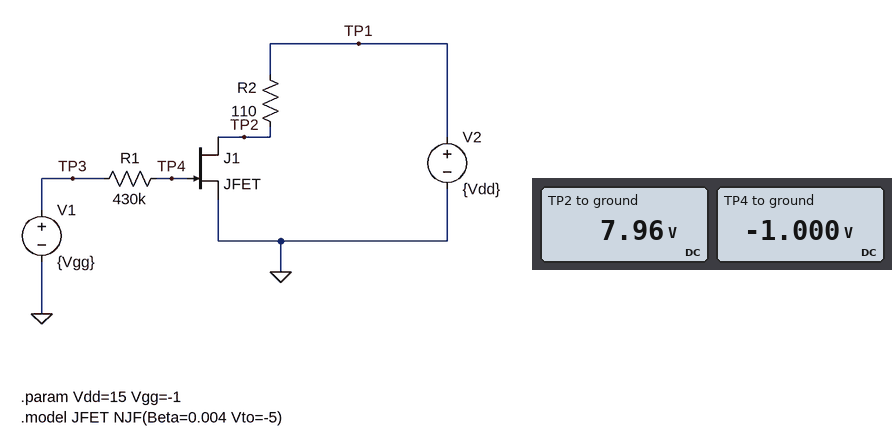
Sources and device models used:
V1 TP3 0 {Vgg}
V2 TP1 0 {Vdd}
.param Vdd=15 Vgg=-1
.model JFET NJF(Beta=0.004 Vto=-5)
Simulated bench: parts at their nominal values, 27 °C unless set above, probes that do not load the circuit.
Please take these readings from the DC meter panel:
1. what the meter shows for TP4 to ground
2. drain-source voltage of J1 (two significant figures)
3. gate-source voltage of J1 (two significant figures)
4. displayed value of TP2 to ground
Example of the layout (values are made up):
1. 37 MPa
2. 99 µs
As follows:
1. -1.000 V
2. 8.0 V
3. -1.0 V
4. 7.96 V
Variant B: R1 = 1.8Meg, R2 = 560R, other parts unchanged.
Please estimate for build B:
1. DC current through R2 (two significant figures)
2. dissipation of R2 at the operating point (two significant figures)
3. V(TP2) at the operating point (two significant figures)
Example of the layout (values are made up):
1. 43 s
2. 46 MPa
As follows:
1. 25 mA
2. 360 mW
3. 890 mV
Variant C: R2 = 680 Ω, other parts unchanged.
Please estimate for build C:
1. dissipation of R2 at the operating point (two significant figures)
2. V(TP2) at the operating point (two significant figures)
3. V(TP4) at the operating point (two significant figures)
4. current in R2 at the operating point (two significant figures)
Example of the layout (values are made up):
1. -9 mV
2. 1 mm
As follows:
1. 300 mW
2. 720 mV
3. -1.0 V
4. 21 mA
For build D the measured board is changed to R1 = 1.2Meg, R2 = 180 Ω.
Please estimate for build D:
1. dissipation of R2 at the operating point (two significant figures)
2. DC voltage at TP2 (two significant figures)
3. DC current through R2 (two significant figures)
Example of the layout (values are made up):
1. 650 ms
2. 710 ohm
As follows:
1. 720 mW
2. 3.6 V
3. 63 mA
